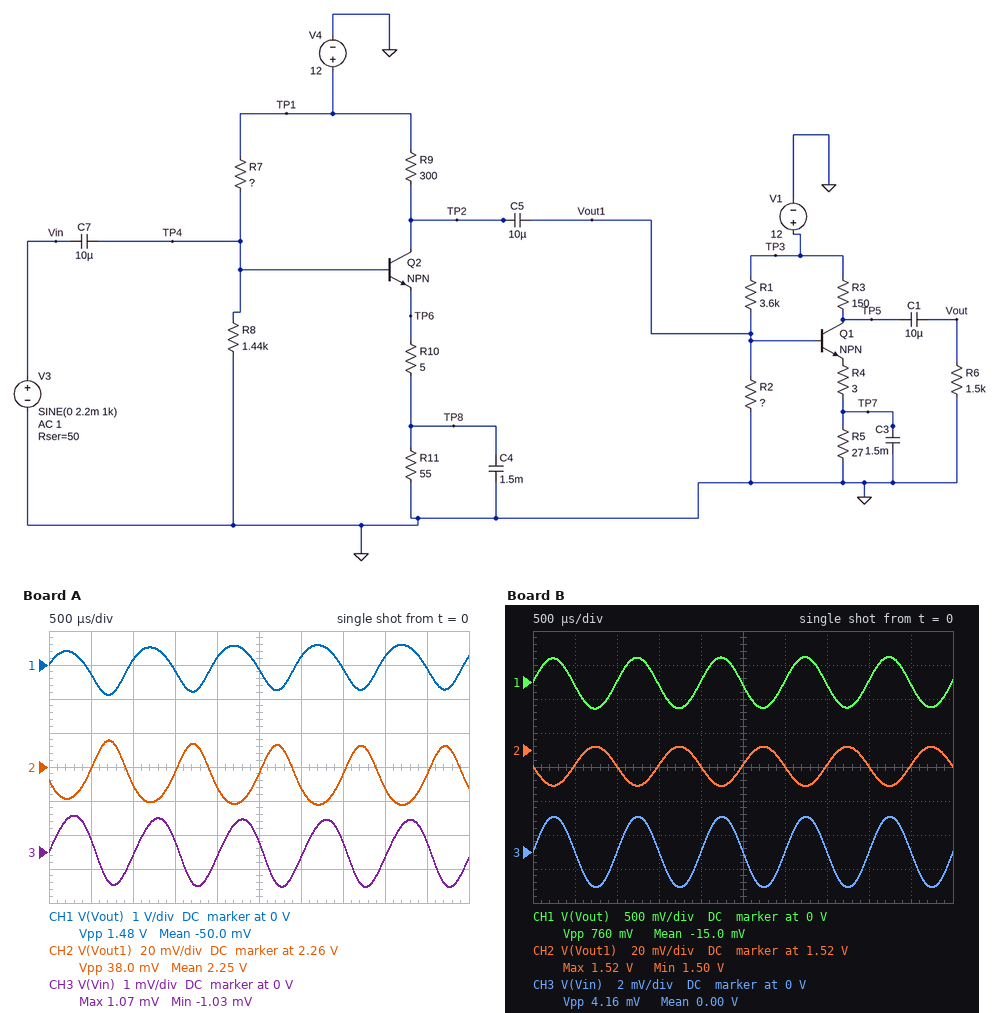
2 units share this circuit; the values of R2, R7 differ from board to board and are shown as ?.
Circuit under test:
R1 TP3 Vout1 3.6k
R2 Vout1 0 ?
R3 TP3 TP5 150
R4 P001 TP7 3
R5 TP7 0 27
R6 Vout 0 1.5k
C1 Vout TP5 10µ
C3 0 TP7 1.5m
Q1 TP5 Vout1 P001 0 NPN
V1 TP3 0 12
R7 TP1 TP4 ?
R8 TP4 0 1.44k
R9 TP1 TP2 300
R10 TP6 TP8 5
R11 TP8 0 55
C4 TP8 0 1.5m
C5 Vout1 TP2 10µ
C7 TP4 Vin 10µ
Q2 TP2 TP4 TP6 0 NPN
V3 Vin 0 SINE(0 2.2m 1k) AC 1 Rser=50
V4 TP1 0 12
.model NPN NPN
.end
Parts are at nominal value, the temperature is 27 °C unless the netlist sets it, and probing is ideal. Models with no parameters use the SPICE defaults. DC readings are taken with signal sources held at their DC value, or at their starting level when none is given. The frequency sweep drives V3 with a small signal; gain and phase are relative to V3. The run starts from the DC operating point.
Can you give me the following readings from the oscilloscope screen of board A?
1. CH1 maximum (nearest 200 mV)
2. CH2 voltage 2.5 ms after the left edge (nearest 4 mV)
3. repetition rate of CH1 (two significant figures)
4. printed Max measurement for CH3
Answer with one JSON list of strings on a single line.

["600 mV", "2.256 V", "1.0 kHz", "1.07 mV"]
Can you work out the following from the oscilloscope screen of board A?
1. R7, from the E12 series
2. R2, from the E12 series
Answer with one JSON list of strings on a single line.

["3.9 kΩ", "1 kΩ"]
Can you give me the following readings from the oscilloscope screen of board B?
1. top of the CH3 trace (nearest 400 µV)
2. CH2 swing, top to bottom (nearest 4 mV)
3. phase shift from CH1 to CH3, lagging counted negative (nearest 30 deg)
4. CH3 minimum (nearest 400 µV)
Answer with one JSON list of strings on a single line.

["2.0 mV", "24 mV", "0 deg", "-2.0 mV"]
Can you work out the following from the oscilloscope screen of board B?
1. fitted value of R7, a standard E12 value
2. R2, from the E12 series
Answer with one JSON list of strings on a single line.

["18 kΩ", "560 Ω"]
